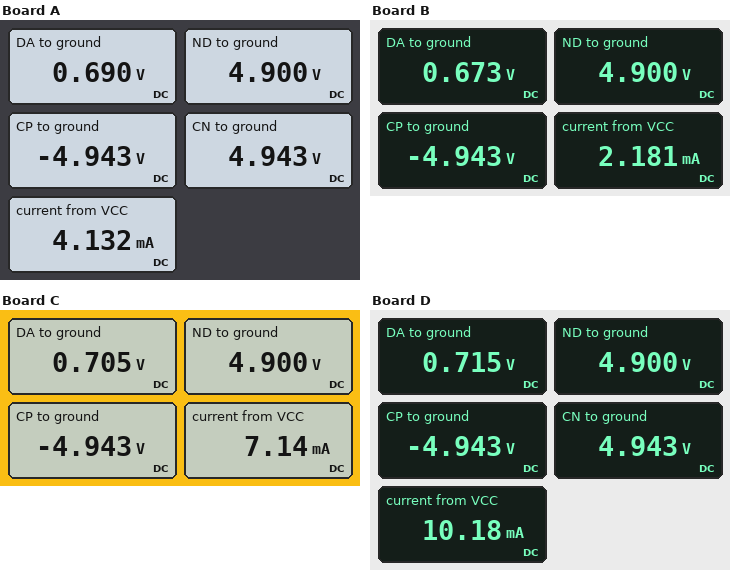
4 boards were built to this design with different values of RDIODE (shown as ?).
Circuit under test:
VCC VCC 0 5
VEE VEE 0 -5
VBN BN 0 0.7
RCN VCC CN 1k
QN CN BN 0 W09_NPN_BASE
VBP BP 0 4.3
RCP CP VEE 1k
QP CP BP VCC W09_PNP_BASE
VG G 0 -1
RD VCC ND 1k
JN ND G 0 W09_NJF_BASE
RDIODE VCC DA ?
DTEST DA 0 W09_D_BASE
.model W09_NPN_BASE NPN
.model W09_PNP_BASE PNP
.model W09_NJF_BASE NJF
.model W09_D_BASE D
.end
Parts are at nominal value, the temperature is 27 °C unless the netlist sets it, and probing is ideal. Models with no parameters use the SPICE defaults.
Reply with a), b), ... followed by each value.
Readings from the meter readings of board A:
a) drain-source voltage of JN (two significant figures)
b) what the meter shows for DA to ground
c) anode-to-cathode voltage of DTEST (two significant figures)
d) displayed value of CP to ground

a) 4.9 V
b) 0.690 V
c) 690 mV
d) -4.943 V
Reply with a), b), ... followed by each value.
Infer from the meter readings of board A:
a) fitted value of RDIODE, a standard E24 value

a) 1.1 kΩ
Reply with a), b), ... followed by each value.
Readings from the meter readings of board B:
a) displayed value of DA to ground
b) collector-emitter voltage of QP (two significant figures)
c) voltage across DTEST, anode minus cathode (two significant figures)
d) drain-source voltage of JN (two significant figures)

a) 0.673 V
b) -9.9 V
c) 670 mV
d) 4.9 V
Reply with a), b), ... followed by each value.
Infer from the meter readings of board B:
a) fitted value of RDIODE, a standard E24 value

a) 2.2 kΩ
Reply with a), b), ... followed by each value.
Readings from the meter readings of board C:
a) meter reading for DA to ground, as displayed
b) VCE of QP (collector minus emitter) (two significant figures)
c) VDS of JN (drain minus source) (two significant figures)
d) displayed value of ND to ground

a) 0.705 V
b) -9.9 V
c) 4.9 V
d) 4.900 V
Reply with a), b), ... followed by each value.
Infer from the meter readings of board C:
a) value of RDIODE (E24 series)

a) 620 Ω
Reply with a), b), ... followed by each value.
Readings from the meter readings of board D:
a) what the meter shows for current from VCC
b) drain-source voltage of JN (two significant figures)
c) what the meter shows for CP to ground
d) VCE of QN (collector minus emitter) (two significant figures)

a) 10.18 mA
b) 4.9 V
c) -4.943 V
d) 4.9 V
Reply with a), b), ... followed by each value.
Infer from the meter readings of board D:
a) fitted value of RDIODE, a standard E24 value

a) 430 Ω
